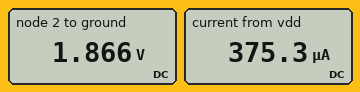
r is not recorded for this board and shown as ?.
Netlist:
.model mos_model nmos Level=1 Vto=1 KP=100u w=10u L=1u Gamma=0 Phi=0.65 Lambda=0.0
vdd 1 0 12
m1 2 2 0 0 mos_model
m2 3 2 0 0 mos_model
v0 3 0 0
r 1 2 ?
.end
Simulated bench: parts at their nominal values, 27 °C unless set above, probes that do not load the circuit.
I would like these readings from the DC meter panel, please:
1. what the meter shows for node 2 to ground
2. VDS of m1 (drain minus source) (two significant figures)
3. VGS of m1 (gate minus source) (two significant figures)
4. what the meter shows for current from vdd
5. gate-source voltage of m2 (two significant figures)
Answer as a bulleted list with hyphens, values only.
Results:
- 1.866 V
- 1.9 V
- 1.9 V
- 375.3 µA
- 1.9 V
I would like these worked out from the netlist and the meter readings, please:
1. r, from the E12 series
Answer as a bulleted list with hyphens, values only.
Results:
- 27 kΩ
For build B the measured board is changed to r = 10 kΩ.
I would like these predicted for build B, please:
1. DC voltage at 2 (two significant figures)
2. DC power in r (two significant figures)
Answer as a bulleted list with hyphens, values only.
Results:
- 2.4 V
- 9.2 mW
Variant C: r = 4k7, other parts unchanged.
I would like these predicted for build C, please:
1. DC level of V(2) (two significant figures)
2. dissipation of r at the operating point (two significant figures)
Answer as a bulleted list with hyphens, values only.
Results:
- 3.0 V
- 17 mW
